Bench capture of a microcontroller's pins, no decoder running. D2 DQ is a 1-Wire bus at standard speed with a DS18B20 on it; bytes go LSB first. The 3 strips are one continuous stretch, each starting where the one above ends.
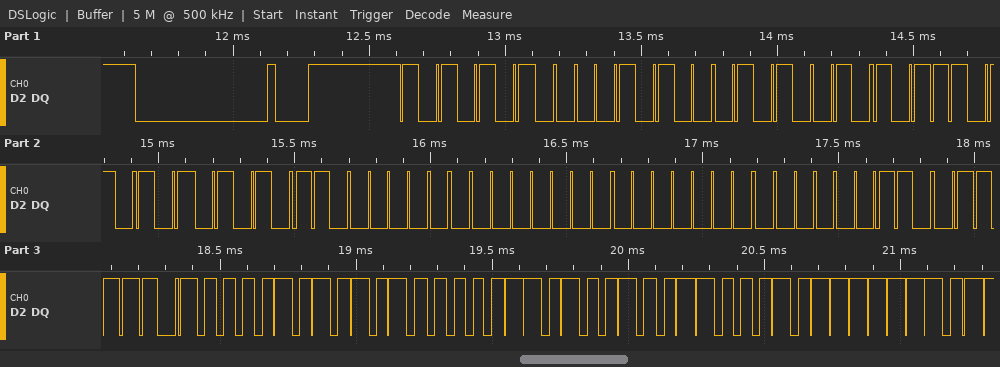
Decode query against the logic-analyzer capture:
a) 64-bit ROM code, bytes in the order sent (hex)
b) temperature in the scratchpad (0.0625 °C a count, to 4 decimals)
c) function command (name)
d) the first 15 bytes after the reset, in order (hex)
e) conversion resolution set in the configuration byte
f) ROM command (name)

28 4A 5D 55 03 00 00 60
85.0000 °C
Read Scratchpad
55 28 4A 5D 55 03 00 00 60 BE 50 05 4B 46 7F
12 bits
Match ROM
